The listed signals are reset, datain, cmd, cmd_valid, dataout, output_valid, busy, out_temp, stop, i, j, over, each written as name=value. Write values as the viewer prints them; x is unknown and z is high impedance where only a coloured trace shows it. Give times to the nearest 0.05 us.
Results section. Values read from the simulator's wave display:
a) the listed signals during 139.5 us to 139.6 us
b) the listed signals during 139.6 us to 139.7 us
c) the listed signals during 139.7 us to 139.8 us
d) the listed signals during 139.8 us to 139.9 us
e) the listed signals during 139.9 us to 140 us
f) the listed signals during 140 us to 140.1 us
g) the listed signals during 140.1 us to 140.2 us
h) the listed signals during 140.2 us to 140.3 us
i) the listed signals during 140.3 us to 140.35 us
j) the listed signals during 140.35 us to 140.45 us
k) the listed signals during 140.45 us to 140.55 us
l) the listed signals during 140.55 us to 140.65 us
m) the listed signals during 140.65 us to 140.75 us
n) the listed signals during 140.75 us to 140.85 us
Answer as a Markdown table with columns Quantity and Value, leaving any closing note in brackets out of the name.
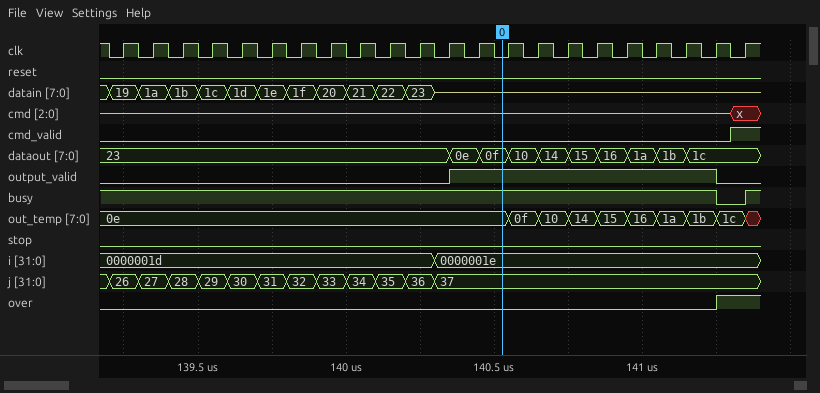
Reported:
| Quantity | Value |
|---|---|
| the listed signals during 139.5 us to 139.6 us | reset=0, datain=1c, cmd=z, cmd_valid=0, dataout=23, output_valid=0, busy=1, out_temp=0e, stop=0, i=0000001d, j=29, over=0 |
| the listed signals during 139.6 us to 139.7 us | reset=0, datain=1d, cmd=z, cmd_valid=0, dataout=23, output_valid=0, busy=1, out_temp=0e, stop=0, i=0000001d, j=30, over=0 |
| the listed signals during 139.7 us to 139.8 us | reset=0, datain=1e, cmd=z, cmd_valid=0, dataout=23, output_valid=0, busy=1, out_temp=0e, stop=0, i=0000001d, j=31, over=0 |
| the listed signals during 139.8 us to 139.9 us | reset=0, datain=1f, cmd=z, cmd_valid=0, dataout=23, output_valid=0, busy=1, out_temp=0e, stop=0, i=0000001d, j=32, over=0 |
| the listed signals during 139.9 us to 140 us | reset=0, datain=20, cmd=z, cmd_valid=0, dataout=23, output_valid=0, busy=1, out_temp=0e, stop=0, i=0000001d, j=33, over=0 |
| the listed signals during 140 us to 140.1 us | reset=0, datain=21, cmd=z, cmd_valid=0, dataout=23, output_valid=0, busy=1, out_temp=0e, stop=0, i=0000001d, j=34, over=0 |
| the listed signals during 140.1 us to 140.2 us | reset=0, datain=22, cmd=z, cmd_valid=0, dataout=23, output_valid=0, busy=1, out_temp=0e, stop=0, i=0000001d, j=35, over=0 |
| the listed signals during 140.2 us to 140.3 us | reset=0, datain=23, cmd=z, cmd_valid=0, dataout=23, output_valid=0, busy=1, out_temp=0e, stop=0, i=0000001d, j=36, over=0 |
| the listed signals during 140.3 us to 140.35 us | reset=0, datain=z, cmd=z, cmd_valid=0, dataout=23, output_valid=0, busy=1, out_temp=0e, stop=0, i=0000001e, j=37, over=0 |
| the listed signals during 140.35 us to 140.45 us | reset=0, datain=z, cmd=z, cmd_valid=0, dataout=0e, output_valid=1, busy=1, out_temp=0e, stop=0, i=0000001e, j=37, over=0 |
| the listed signals during 140.45 us to 140.55 us | reset=0, datain=z, cmd=z, cmd_valid=0, dataout=0f, output_valid=1, busy=1, out_temp=0e, stop=0, i=0000001e, j=37, over=0 |
| the listed signals during 140.55 us to 140.65 us | reset=0, datain=z, cmd=z, cmd_valid=0, dataout=10, output_valid=1, busy=1, out_temp=0f, stop=0, i=0000001e, j=37, over=0 |
| the listed signals during 140.65 us to 140.75 us | reset=0, datain=z, cmd=z, cmd_valid=0, dataout=14, output_valid=1, busy=1, out_temp=10, stop=0, i=0000001e, j=37, over=0 |
| the listed signals during 140.75 us to 140.85 us | reset=0, datain=z, cmd=z, cmd_valid=0, dataout=15, output_valid=1, busy=1, out_temp=14, stop=0, i=0000001e, j=37, over=0 |
